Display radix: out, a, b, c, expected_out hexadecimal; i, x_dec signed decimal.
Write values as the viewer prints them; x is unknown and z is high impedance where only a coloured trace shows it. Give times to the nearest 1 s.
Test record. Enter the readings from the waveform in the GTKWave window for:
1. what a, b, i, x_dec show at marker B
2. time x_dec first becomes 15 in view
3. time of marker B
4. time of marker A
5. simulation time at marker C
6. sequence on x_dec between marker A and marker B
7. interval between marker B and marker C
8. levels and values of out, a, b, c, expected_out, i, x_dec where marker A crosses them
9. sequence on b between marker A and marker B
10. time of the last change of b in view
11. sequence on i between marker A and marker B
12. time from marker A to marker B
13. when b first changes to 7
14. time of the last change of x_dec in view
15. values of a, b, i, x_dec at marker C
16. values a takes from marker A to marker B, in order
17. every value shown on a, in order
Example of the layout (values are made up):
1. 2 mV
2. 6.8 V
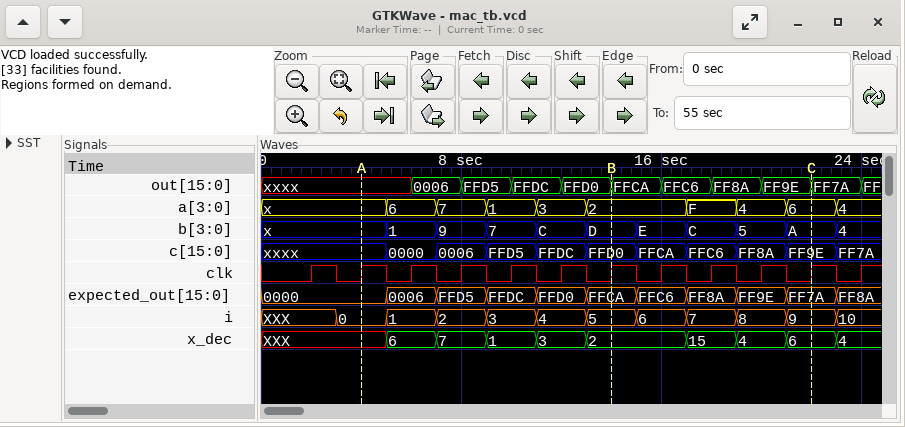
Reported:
1. a=2, b=D, i=5, x_dec=2
2. 17 s
3. 14 s
4. 4 s
5. 22 s
6. XXX, 6, 7, 1, 3, 2
7. 8 s
8. out=xxxx, a=x, b=x, c=xxxx, expected_out=0000, i=0, x_dec=XXX
9. x, 1, 9, 7, C, D
10. 23 s
11. 0, 1, 2, 3, 4, 5
12. 10 s
13. 9 s
14. 23 s
15. a=6, b=A, i=9, x_dec=6
16. x, 6, 7, 1, 3, 2
17. x, 6, 7, 1, 3, 2, F, 4, 6, 4
